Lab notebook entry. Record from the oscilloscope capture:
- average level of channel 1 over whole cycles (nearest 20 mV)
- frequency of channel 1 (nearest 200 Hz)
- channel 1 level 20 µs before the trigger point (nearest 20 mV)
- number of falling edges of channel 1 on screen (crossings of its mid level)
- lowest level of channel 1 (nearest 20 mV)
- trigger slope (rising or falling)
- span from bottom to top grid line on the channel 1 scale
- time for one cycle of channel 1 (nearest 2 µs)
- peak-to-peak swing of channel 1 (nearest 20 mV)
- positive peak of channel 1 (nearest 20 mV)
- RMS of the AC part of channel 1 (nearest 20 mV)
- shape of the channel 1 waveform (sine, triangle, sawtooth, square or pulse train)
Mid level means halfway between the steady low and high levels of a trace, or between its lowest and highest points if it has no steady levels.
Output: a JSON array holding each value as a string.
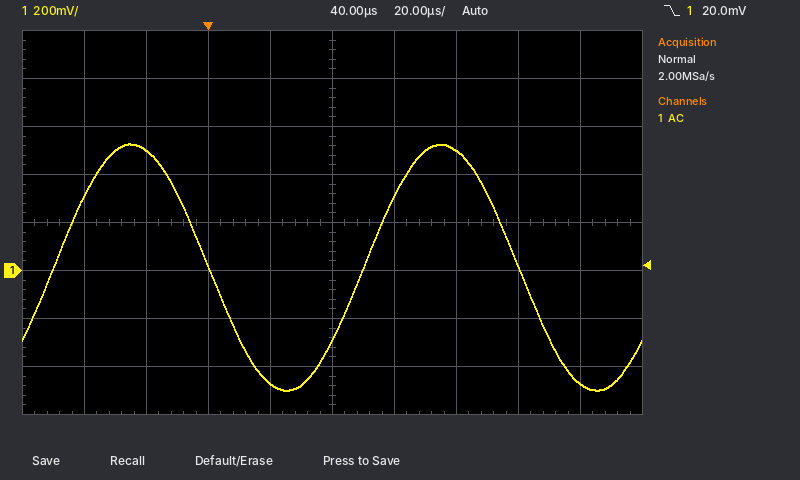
["20 mV", "10.0 kHz", "500 mV", "2", "-500 mV", "falling", "1.6 V", "100 µs", "1.02 V", "520 mV", "360 mV", "sine"]
